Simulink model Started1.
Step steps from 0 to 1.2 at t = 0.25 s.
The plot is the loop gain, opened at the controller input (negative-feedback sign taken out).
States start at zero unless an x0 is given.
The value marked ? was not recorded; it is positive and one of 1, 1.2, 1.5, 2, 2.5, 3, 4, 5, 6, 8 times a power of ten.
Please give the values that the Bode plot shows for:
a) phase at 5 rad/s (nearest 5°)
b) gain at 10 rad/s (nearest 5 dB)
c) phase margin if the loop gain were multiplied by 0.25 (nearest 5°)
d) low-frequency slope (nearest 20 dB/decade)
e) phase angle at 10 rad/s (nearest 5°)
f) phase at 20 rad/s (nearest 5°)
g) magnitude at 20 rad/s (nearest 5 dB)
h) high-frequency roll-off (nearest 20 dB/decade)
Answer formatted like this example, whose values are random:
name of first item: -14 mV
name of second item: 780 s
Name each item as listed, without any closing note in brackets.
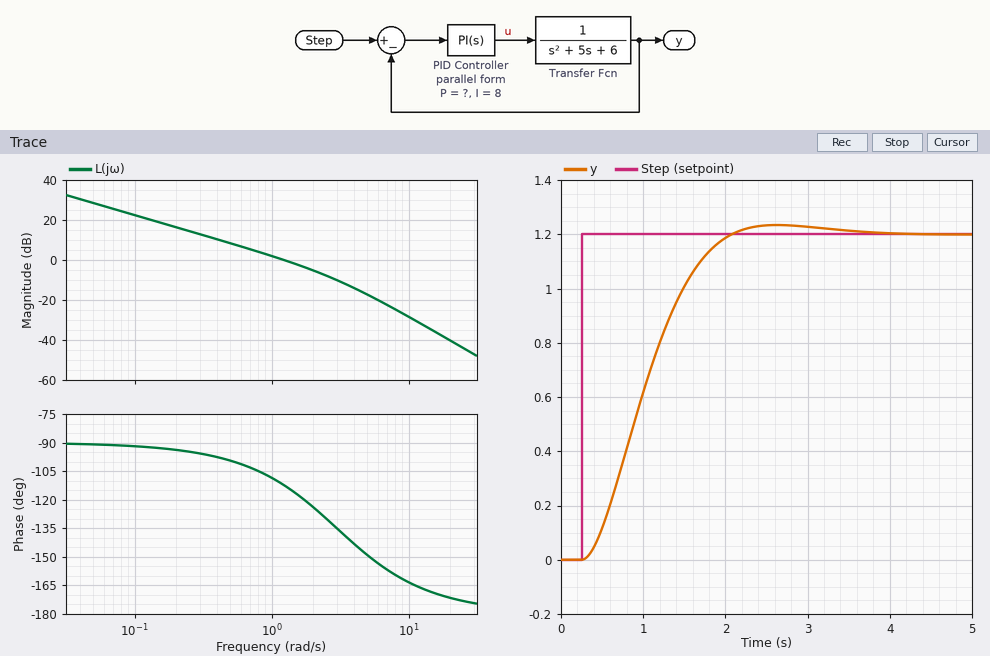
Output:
phase at 5 rad/s: -150°
gain at 10 rad/s: -30 dB
phase margin if the loop gain were multiplied by 0.25: 85°
low-frequency slope: -20 dB/decade
phase angle at 10 rad/s: -165°
phase at 20 rad/s: -170°
magnitude at 20 rad/s: -40 dB
high-frequency roll-off: -40 dB/decade
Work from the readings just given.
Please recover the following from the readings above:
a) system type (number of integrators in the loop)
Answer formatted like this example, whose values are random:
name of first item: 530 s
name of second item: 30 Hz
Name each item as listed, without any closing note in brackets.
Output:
system type: 1
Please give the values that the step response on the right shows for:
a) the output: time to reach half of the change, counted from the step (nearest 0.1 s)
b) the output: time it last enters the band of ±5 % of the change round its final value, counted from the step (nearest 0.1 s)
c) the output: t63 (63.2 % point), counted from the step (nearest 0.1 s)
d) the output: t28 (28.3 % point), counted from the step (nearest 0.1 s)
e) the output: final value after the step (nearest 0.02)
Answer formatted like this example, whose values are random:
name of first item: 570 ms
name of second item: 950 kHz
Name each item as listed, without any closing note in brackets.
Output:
the output: time to reach half of the change, counted from the step: 0.7 s
the output: time it last enters the band of ±5 % of the change round its final value, counted from the step: 1.6 s
the output: t63 (63.2 % point), counted from the step: 0.9 s
the output: t28 (28.3 % point), counted from the step: 0.5 s
the output: final value after the step: 1.20
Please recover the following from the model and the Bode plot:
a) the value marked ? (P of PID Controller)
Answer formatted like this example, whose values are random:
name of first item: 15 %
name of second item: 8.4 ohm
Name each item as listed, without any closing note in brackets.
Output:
the value marked ?: 4
